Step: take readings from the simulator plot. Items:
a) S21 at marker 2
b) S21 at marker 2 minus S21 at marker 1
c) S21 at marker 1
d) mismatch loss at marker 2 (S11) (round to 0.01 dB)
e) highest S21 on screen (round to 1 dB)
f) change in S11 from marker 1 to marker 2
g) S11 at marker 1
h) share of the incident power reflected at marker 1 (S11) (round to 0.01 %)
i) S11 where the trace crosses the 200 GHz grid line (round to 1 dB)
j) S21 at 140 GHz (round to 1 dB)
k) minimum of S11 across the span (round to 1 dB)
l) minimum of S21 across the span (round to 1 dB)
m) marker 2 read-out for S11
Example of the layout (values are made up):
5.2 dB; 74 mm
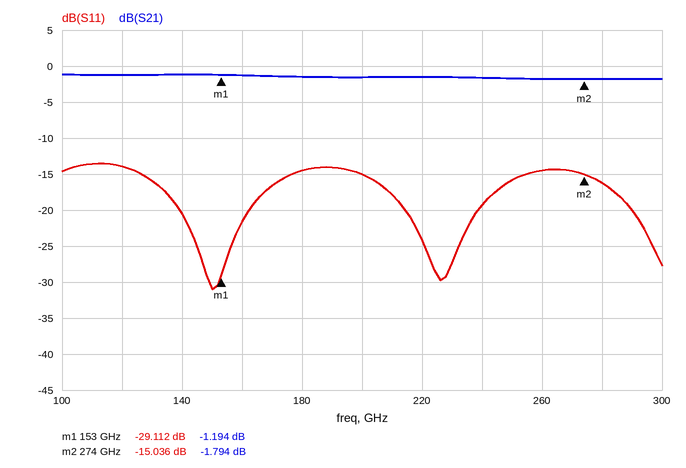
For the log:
-1.794 dB; -0.600 dB; -1.194 dB; 0.14 dB; -1 dB; 14.076 dB; -29.112 dB; 0.12 %; -15 dB; -1 dB; -31 dB; -2 dB; -15.036 dB
